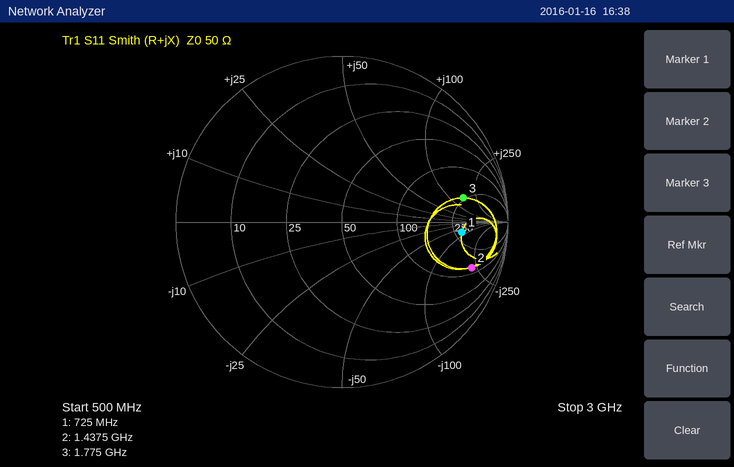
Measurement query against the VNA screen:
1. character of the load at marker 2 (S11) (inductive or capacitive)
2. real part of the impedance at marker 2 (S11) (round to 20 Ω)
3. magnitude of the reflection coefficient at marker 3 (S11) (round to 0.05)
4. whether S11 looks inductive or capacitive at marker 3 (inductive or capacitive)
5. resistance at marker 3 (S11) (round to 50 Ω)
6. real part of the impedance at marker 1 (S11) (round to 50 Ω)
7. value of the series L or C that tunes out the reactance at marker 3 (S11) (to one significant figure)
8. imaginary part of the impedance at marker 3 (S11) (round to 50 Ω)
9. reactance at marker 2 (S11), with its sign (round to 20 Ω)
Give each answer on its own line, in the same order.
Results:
capacitive
120 Ω
0.75
inductive
250 Ω
300 Ω
600 fF
+150 Ω
-220 Ω
